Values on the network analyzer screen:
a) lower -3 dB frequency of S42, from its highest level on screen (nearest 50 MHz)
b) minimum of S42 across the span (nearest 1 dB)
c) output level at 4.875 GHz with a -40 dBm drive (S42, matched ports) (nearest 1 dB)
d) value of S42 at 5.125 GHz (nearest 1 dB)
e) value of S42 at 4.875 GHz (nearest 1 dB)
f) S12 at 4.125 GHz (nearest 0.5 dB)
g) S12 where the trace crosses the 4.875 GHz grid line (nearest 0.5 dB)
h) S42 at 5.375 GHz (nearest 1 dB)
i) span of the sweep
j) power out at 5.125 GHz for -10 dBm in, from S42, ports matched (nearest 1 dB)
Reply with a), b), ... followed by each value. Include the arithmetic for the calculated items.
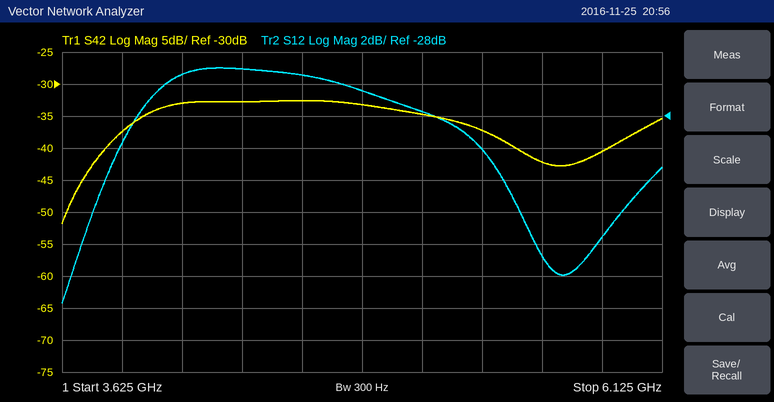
a) 3.95 GHz
b) -52 dB
c) -40 dBm + (-33 dB) = -73 dBm
d) -35 dB
e) -33 dB
f) -25.5 dB
g) -26.5 dB
h) -37 dB
i) 2.5 GHz
j) -10 dBm + (-35 dB) = -45 dBm
